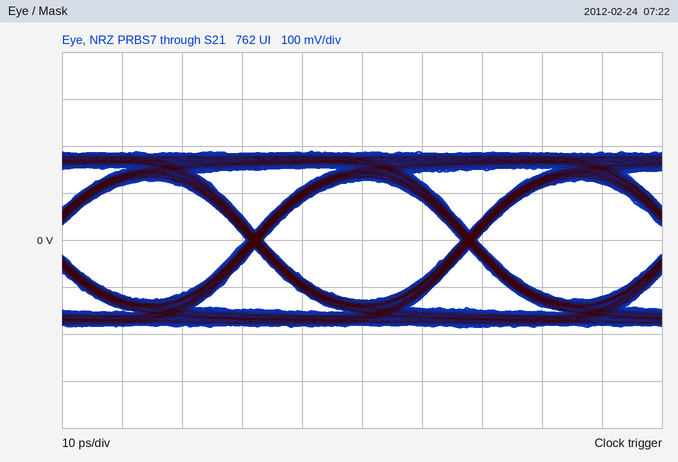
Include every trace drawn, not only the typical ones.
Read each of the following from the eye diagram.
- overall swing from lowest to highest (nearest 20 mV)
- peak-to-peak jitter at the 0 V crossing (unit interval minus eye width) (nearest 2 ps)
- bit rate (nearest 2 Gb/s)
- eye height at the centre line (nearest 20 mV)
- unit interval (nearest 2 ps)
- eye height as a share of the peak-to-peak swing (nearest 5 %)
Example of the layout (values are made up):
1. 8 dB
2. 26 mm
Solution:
1. 380 mV
2. 2 ps
3. 28 Gb/s
4. 260 mV
5. 36 ps
6. 70 %
